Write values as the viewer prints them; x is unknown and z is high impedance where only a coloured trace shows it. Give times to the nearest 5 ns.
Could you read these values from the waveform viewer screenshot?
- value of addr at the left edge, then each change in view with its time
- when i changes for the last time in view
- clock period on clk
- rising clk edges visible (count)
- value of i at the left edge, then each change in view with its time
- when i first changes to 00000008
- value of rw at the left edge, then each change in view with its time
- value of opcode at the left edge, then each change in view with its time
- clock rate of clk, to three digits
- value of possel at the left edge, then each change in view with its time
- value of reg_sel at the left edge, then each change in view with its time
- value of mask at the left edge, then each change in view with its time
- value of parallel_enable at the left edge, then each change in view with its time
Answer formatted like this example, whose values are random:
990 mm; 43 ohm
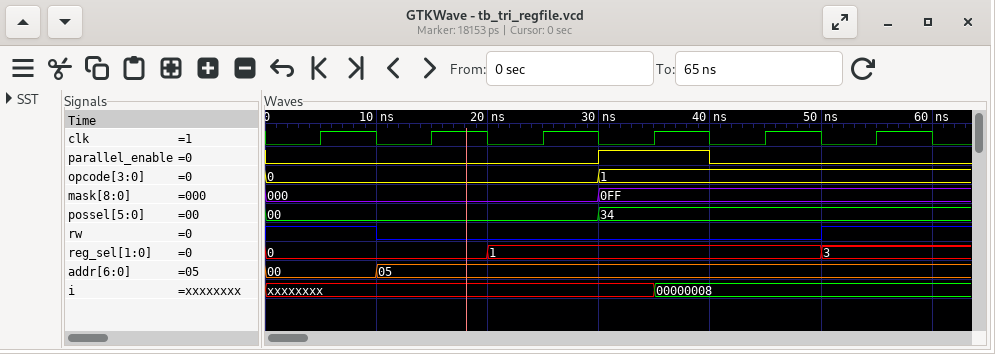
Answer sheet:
00, 05 at 10 ns; 35 ns; 10 ns; 6; xxxxxxxx, 00000008 at 35 ns; 35 ns; 1, 0 at 10 ns, 1 at 50 ns; 0, 1 at 30 ns; 100 MHz; 00, 34 at 30 ns; 0, 1 at 20 ns, 3 at 50 ns; 000, 0FF at 30 ns; 0, 1 at 30 ns, 0 at 40 ns
